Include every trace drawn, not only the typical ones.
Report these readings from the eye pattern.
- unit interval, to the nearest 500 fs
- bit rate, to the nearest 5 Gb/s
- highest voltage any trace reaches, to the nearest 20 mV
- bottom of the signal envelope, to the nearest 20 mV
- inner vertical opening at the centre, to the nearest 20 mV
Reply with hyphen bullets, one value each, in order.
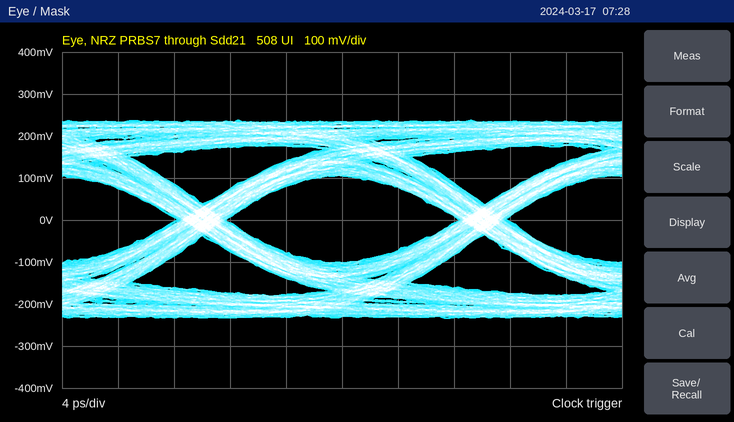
- 20.0 ps
- 50 Gb/s
- 240 mV
- -240 mV
- 200 mV
